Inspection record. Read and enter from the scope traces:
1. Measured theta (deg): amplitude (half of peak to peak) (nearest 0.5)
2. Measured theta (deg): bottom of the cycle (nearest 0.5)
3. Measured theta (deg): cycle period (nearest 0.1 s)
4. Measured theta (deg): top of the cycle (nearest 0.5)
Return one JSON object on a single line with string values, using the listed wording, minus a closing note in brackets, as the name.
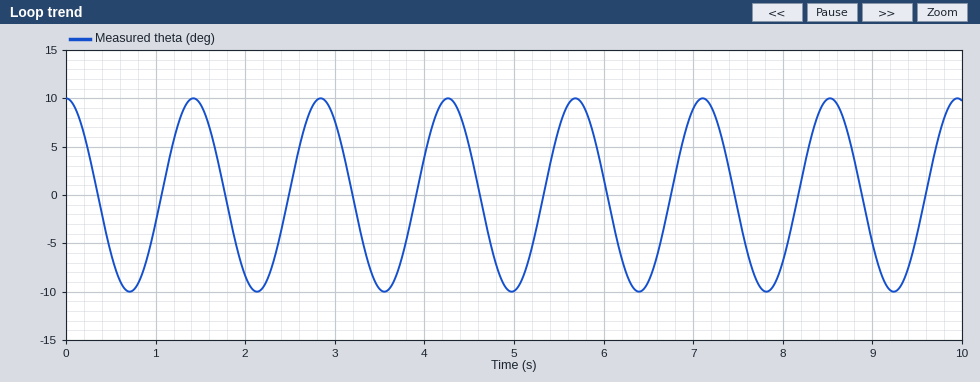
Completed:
{"Measured theta (deg): amplitude (half of peak to peak)": "10.0", "Measured theta (deg): bottom of the cycle": "-10.0", "Measured theta (deg): cycle period": "1.4 s", "Measured theta (deg): top of the cycle": "10.0"}
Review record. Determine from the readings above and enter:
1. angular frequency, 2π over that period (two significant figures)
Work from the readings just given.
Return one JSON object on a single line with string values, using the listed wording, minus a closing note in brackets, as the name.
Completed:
{"angular frequency, 2π over that period": "4.5 rad/s"}
